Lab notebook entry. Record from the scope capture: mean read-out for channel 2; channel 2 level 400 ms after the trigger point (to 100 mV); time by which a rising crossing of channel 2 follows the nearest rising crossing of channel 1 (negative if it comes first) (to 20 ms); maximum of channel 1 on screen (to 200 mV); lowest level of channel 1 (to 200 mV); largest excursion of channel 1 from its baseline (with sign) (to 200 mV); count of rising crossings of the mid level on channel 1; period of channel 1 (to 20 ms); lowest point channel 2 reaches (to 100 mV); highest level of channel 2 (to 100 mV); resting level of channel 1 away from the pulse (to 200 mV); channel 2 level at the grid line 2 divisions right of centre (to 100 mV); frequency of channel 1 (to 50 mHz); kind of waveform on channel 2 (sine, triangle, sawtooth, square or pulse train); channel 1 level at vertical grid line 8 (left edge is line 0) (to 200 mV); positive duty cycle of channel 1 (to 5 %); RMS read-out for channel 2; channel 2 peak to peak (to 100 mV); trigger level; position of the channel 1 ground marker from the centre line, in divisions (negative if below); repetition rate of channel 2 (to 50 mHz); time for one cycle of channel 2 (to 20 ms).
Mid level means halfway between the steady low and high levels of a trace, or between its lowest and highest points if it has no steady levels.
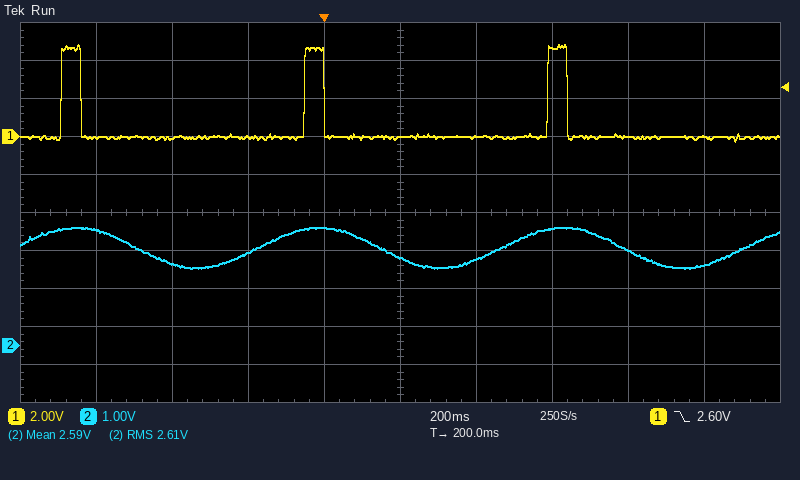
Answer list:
2.59 V
2.3 V
-120 ms
4.8 V
-200 mV
+4.8 V
3
640 ms
2.0 V
3.1 V
0.0 V
3.1 V
1.55 Hz
sine
0.0 V
10 %
2.61 V
1.1 V
2.60 V
+2.0 div
1.55 Hz
640 ms
